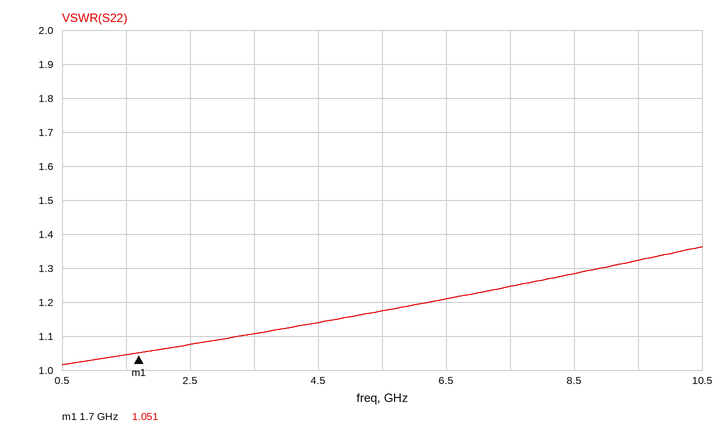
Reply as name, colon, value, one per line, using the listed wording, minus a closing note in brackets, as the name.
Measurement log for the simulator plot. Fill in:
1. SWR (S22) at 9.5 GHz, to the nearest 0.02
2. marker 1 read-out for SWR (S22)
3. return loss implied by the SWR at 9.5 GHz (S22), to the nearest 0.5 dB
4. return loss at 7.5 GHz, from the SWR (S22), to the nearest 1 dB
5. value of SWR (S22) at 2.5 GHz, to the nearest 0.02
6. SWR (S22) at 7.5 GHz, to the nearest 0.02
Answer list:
SWR (S22) at 9.5 GHz, to the nearest 0.02: 1.32
marker 1 read-out for SWR: 1.051
return loss implied by the SWR at 9.5 GHz (S22), to the nearest 0.5 dB: 17.0 dB
return loss at 7.5 GHz, from the SWR (S22), to the nearest 1 dB: 19 dB
value of SWR (S22) at 2.5 GHz, to the nearest 0.02: 1.08
SWR (S22) at 7.5 GHz, to the nearest 0.02: 1.24
